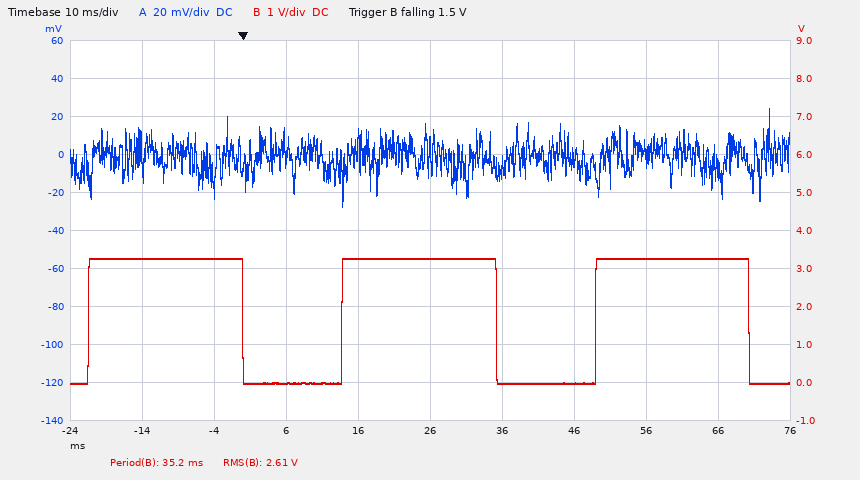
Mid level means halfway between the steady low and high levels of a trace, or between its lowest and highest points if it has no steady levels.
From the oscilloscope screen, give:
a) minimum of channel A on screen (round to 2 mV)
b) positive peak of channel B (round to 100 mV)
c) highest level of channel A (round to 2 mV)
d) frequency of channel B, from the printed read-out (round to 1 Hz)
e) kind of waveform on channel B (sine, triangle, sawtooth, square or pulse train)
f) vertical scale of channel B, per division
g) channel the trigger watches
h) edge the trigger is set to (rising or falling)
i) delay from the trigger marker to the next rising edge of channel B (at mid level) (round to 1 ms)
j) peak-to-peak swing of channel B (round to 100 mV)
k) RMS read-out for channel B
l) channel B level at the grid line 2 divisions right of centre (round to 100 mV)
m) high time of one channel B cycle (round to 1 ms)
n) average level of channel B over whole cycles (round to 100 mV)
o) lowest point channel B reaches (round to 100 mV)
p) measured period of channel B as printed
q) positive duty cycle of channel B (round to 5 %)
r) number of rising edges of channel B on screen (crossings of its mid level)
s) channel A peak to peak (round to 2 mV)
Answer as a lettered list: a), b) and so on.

a) -28 mV
b) 3.3 V
c) 24 mV
d) 28 Hz
e) pulse train
f) 1 V
g) channel B
h) falling
i) 14 ms
j) 3.3 V
k) 2.61 V
l) 0.0 V
m) 21 ms
n) 2.0 V
o) 0.0 V
p) 35.2 ms
q) 60 %
r) 3
s) 52 mV
